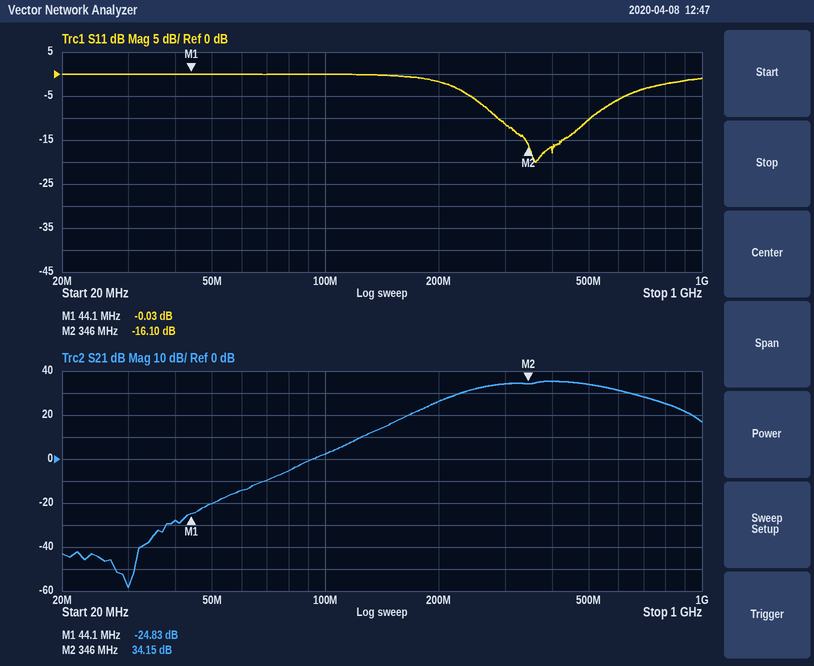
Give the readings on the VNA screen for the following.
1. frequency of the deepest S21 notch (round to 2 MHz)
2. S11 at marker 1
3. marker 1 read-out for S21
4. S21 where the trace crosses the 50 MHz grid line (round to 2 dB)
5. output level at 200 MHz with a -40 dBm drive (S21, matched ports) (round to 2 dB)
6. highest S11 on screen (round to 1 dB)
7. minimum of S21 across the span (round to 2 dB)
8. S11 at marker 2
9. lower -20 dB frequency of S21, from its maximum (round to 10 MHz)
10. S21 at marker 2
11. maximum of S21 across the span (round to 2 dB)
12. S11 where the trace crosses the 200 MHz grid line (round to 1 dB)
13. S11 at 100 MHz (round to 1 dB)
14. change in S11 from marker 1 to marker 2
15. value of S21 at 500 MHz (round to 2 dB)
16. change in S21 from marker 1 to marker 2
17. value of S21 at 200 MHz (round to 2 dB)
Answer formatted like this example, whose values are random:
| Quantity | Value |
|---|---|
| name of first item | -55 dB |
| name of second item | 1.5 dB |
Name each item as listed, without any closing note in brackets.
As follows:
| Quantity | Value |
|---|---|
| frequency of the deepest S21 notch | 30 MHz |
| S11 at marker 1 | -0.03 dB |
| marker 1 read-out for S21 | -24.83 dB |
| S21 where the trace crosses the 50 MHz grid line | -20 dB |
| output level at 200 MHz with a -40 dBm drive (S21, matched ports) | -14 dBm |
| highest S11 on screen | 0 dB |
| minimum of S21 across the span | -58 dB |
| S11 at marker 2 | -16.10 dB |
| lower -20 dB frequency of S21, from its maximum | 150 MHz |
| S21 at marker 2 | 34.15 dB |
| maximum of S21 across the span | 36 dB |
| S11 where the trace crosses the 200 MHz grid line | -2 dB |
| S11 at 100 MHz | 0 dB |
| change in S11 from marker 1 to marker 2 | -16.07 dB |
| value of S21 at 500 MHz | 34 dB |
| change in S21 from marker 1 to marker 2 | 58.98 dB |
| value of S21 at 200 MHz | 26 dB |
